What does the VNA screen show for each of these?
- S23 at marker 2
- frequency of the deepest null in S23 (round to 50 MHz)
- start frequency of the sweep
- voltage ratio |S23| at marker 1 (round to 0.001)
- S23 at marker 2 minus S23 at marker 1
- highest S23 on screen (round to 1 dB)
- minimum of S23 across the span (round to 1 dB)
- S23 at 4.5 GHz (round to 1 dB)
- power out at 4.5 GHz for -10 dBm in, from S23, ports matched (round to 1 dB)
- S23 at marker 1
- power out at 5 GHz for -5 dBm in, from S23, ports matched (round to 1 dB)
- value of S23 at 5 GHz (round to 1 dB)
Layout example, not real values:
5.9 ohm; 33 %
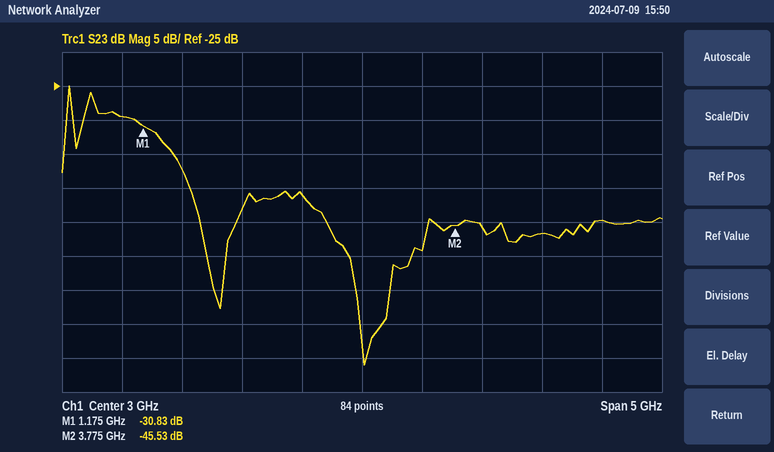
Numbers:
-45.53 dB; 3.00 GHz; 500 MHz; 0.029; -14.70 dB; -25 dB; -66 dB; -47 dB; -57 dBm; -30.83 dB; -50 dBm; -45 dB
